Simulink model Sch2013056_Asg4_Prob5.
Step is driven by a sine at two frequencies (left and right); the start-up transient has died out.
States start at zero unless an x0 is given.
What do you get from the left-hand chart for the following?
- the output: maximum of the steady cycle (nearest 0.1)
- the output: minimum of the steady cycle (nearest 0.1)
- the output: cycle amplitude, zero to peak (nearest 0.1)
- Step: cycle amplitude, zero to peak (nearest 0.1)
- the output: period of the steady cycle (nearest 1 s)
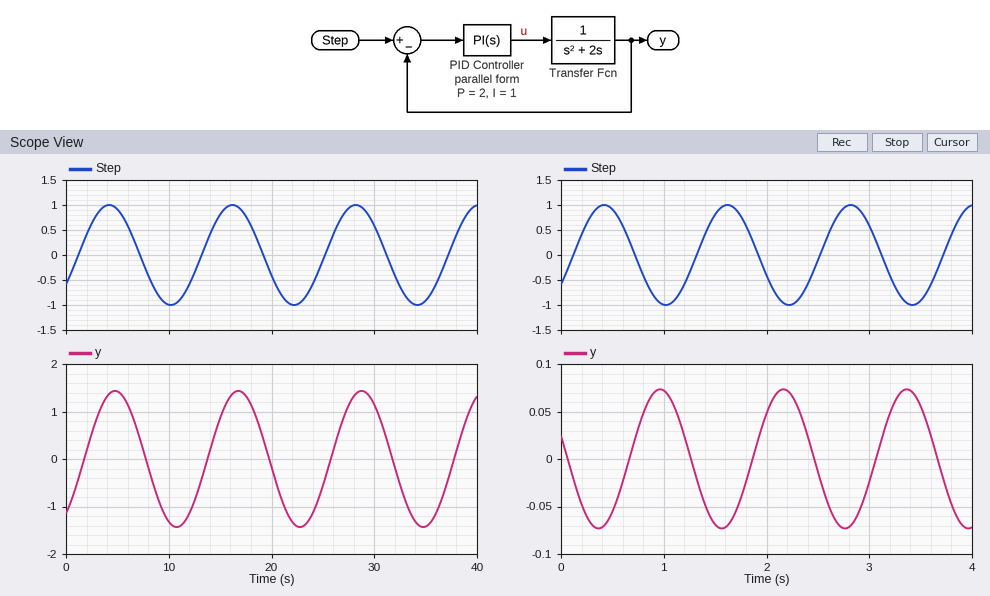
1.4
-1.4
1.4
1.0
12 s
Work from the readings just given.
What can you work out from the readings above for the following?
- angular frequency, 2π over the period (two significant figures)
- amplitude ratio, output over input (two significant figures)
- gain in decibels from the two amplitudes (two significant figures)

0.52 rad/s
1.4
2.9 dB
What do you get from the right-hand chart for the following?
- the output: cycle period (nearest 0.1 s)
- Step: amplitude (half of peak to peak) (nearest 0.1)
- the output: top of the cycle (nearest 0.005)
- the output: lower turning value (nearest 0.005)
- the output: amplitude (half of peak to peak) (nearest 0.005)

1.2 s
1.0
0.075
-0.075
0.075
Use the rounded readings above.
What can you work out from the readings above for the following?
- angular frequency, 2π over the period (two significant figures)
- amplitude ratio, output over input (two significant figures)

5.2 rad/s
0.075
